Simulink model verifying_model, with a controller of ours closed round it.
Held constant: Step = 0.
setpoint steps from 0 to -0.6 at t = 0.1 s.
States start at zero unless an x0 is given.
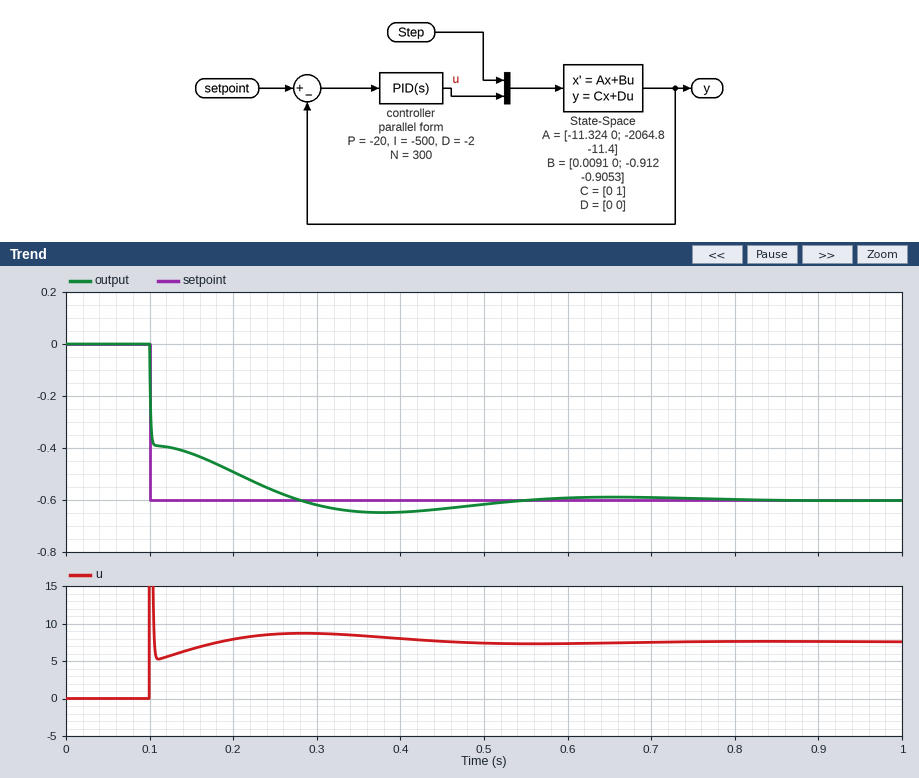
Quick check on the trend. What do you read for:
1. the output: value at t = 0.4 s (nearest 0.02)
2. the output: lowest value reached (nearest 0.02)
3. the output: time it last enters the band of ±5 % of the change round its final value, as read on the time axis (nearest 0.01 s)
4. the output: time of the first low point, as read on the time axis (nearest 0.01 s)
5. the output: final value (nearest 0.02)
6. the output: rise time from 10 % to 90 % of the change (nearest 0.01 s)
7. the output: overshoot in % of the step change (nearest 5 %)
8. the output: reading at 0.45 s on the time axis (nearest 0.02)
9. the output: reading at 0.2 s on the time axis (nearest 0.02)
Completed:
-0.64
-0.64
0.46 s
0.38 s
-0.60
0.13 s
10 %
-0.64
-0.50
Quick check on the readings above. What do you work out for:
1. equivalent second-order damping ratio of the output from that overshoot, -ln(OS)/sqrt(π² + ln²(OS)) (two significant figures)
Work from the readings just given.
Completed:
0.59
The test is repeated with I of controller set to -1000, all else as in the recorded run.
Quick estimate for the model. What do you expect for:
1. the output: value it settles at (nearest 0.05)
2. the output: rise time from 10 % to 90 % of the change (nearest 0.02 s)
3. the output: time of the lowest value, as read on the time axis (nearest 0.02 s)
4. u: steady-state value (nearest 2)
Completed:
-0.60
0.08 s
0.28 s
8
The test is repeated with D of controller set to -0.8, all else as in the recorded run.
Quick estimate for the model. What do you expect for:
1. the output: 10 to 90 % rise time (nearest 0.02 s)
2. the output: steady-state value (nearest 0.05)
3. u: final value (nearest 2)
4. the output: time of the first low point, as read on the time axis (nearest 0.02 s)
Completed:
0.10 s
-0.60
8
0.30 s
